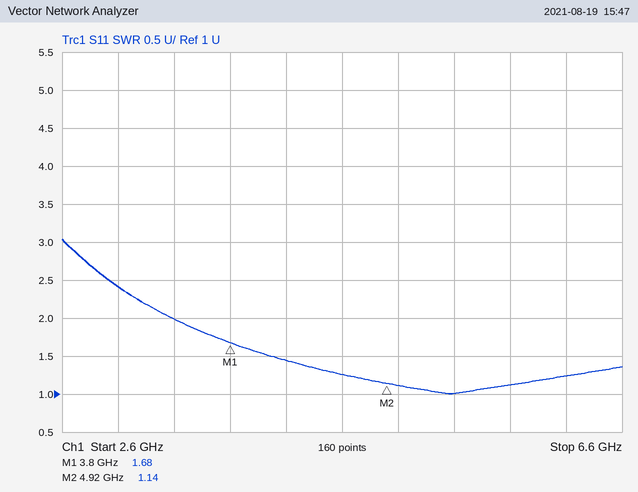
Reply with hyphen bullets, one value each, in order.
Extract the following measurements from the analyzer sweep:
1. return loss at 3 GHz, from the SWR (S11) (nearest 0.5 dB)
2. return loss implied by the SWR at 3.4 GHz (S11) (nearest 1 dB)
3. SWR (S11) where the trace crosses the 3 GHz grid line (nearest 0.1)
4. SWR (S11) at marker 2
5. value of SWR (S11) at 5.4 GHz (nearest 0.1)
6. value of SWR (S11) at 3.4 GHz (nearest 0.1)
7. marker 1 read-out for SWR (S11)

- 7.5 dB
- 10 dB
- 2.4
- 1.14
- 1.0
- 2.0
- 1.68
